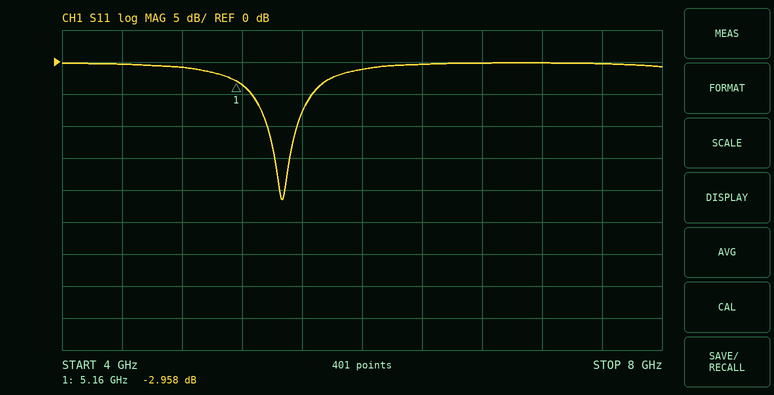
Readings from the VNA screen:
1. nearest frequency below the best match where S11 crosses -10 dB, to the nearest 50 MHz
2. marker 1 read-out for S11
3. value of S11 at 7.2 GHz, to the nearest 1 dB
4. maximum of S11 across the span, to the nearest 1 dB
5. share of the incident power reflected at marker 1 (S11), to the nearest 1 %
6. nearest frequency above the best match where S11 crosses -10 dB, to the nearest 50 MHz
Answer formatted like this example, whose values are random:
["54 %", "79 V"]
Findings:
["5.35 GHz", "-2.958 dB", "0 dB", "0 dB", "51 %", "5.55 GHz"]
